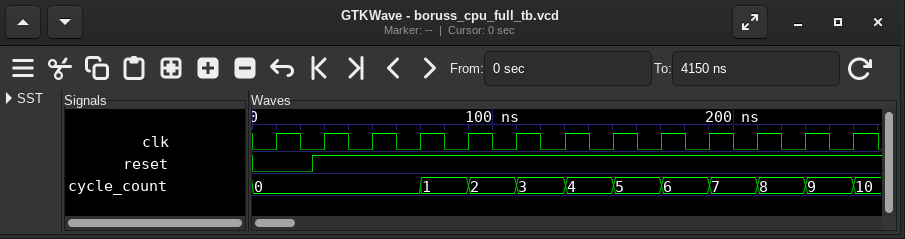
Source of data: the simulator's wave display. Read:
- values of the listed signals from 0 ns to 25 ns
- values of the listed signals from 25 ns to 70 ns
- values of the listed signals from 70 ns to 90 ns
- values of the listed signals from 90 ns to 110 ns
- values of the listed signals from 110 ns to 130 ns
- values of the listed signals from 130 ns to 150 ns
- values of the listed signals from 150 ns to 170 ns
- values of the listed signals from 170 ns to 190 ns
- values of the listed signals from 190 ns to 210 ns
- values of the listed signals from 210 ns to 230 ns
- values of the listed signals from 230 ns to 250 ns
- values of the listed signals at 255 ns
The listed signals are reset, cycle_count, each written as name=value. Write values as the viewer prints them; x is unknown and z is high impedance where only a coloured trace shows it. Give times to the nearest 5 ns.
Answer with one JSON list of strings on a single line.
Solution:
["reset=0, cycle_count=0", "reset=1, cycle_count=0", "reset=1, cycle_count=1", "reset=1, cycle_count=2", "reset=1, cycle_count=3", "reset=1, cycle_count=4", "reset=1, cycle_count=5", "reset=1, cycle_count=6", "reset=1, cycle_count=7", "reset=1, cycle_count=8", "reset=1, cycle_count=9", "reset=1, cycle_count=10"]
